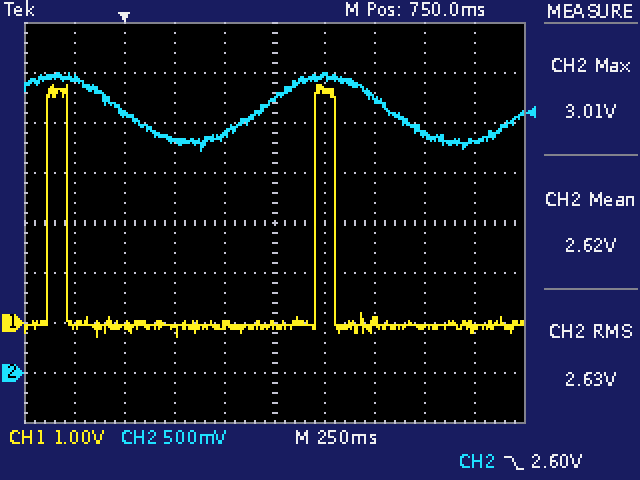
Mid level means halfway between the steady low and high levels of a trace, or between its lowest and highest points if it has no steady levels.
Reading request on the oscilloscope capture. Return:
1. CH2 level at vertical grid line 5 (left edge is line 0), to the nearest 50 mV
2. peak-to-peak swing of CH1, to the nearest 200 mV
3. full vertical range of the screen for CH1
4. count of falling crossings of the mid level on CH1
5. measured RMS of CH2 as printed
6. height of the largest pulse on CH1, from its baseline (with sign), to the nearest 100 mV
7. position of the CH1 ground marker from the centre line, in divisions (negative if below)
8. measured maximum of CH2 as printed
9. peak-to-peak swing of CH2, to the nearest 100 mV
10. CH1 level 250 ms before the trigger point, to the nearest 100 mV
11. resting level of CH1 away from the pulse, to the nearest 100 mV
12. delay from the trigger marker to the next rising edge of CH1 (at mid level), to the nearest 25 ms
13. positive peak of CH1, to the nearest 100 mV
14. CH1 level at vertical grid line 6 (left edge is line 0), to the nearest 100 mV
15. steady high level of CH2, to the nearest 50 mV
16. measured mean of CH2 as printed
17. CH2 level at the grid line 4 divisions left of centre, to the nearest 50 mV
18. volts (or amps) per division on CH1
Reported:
2.75 V
5.0 V
8 V
2
2.63 V
+4.8 V
-2.0 div
3.01 V
800 mV
0.0 V
0.0 V
950 ms
4.8 V
4.7 V
2.95 V
2.62 V
2.95 V
1 V
